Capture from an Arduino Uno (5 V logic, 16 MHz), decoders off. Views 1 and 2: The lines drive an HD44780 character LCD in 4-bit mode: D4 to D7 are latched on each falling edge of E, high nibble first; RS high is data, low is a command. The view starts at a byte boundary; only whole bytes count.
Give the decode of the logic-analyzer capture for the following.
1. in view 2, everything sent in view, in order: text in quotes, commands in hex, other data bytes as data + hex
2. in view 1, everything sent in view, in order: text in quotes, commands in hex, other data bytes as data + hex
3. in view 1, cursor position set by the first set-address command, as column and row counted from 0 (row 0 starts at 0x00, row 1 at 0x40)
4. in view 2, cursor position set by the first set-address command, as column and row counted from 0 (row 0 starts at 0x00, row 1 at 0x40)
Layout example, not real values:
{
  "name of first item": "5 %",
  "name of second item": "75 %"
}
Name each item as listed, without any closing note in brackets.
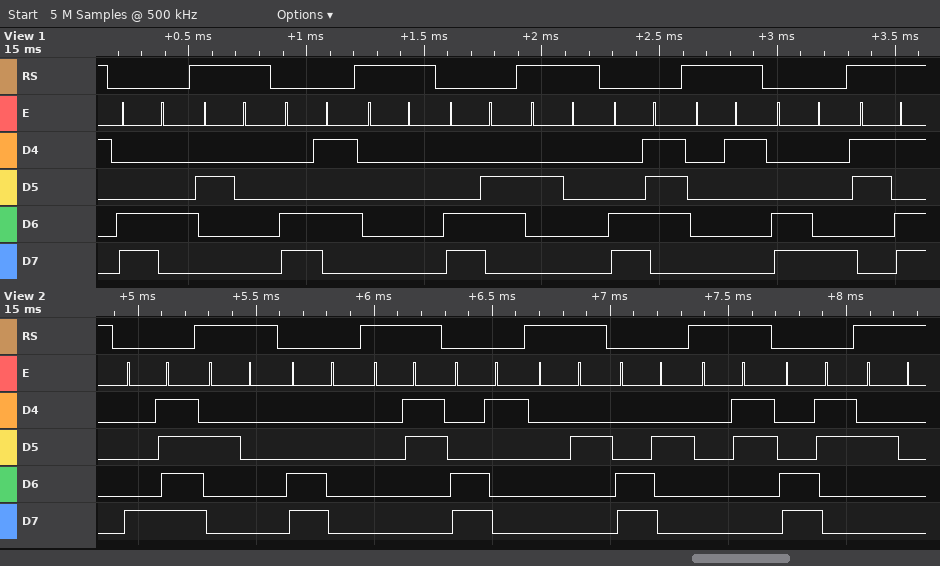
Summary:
{
  "in view 2, everything sent in view, in order: text in quotes, commands in hex, other data bytes as data + hex": "0x8F \" \" 0xC0 data 03 0xC1 data 02 0xC2 data 03 0xC3 \" \"",
  "in view 1, everything sent in view, in order: text in quotes, commands in hex, other data bytes as data + hex": "0xC4 \" \" 0xC5 data 00 0xC6 \" \" 0xC7 data 01 0xC8 \"=\"",
  "in view 1, cursor position set by the first set-address command, as column and row counted from 0": "column 4, row 1",
  "in view 2, cursor position set by the first set-address command, as column and row counted from 0": "column 15, row 0"
}
